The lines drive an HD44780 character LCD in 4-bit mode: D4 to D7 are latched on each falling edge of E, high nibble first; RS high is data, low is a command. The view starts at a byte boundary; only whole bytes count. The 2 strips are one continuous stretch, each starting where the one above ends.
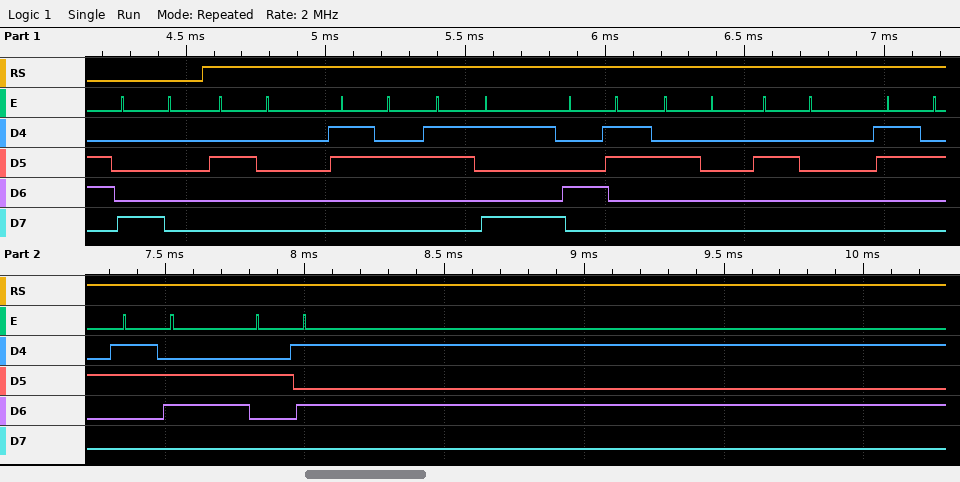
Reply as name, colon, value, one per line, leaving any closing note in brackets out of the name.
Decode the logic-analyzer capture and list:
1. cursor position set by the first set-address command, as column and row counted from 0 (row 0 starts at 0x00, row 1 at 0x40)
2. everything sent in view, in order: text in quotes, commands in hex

cursor position set by the first set-address command, as column and row counted from 0: column 0, row 0
everything sent in view, in order: text in quotes, commands in hex: 0x80 " 29C  26%"
